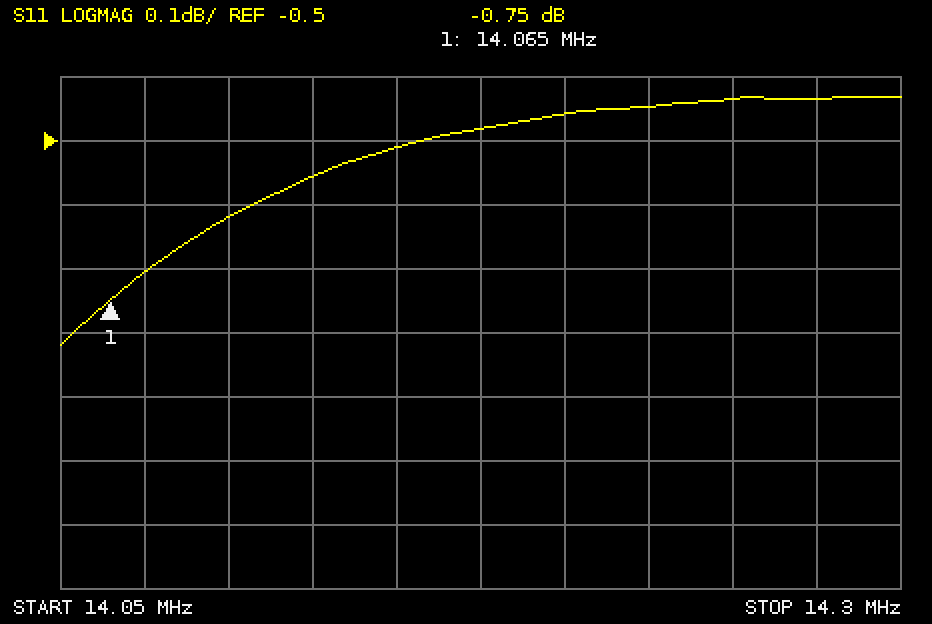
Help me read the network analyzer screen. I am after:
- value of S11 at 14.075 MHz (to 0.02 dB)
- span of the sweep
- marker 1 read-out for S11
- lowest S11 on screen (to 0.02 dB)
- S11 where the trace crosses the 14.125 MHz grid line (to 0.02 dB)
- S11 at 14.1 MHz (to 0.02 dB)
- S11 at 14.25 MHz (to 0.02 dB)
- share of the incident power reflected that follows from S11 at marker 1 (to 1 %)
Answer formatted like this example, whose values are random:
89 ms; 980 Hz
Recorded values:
-0.70 dB; 250 kHz; -0.75 dB; -0.82 dB; -0.56 dB; -0.62 dB; -0.44 dB; 84 %
